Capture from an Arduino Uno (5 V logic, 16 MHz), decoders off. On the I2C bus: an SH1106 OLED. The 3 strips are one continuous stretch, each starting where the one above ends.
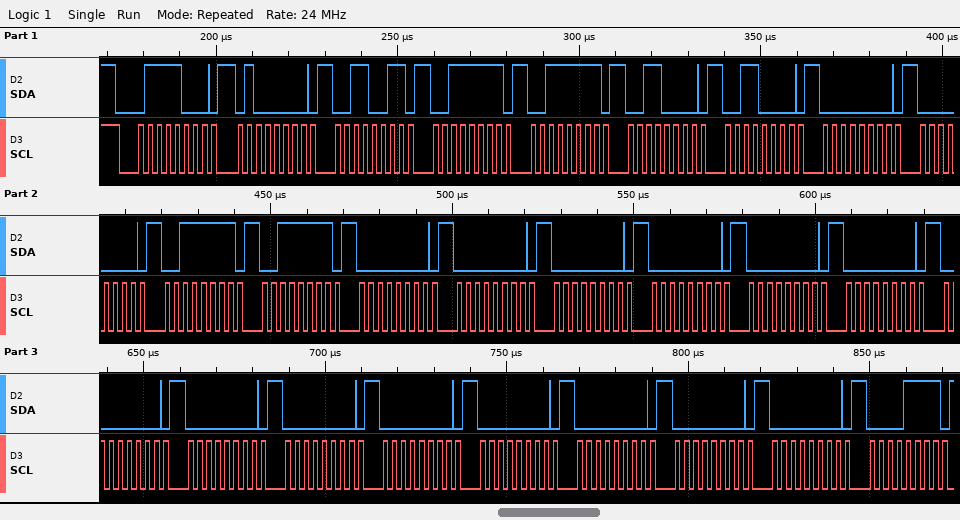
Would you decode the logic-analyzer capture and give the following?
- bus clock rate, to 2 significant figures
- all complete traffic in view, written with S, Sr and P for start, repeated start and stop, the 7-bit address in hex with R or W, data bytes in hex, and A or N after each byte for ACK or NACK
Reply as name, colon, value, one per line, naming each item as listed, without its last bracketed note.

bus clock rate, to 2 significant figures: 400 kHz
all complete traffic in view, written with S, Sr and P for start, repeated start and stop, the 7-bit address in hex with R or W, data bytes in hex, and A or N after each byte for ACK or NACK: S 3CW A 40 A 33 A 3F A 3F A 30 A 30 A 00 A 00 A 3F A 3F A 00 A 00 A 00 A 00 A 00 A 00 A 00 A 00 A 00 A 00 A 00 A 00 A 00 A 00 A 0F A
